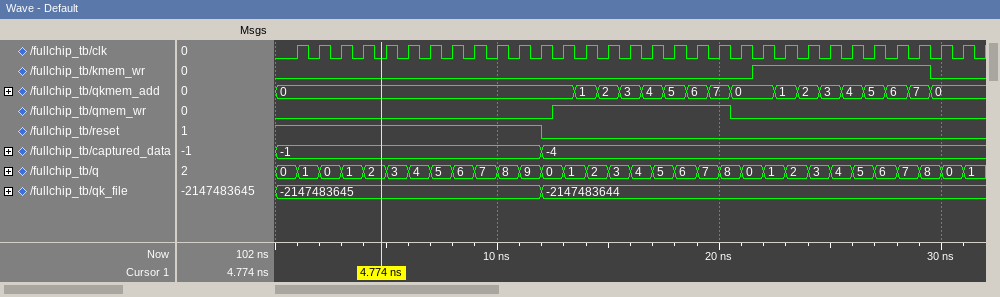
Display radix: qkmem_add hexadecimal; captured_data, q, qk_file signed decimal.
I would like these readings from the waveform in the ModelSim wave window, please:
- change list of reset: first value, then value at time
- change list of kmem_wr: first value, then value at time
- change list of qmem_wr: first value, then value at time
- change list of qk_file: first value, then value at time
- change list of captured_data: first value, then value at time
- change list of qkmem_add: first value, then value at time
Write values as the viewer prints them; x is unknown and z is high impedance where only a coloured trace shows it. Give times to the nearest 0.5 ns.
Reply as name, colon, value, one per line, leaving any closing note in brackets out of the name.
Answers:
change list of reset: first value, then value at time: 1, 0 at 12 ns
change list of kmem_wr: first value, then value at time: 0, 1 at 21.5 ns, 0 at 29.5 ns
change list of qmem_wr: first value, then value at time: 0, 1 at 12.5 ns, 0 at 20.5 ns
change list of qk_file: first value, then value at time: -2147483645, -2147483644 at 12 ns
change list of captured_data: first value, then value at time: -1, -4 at 12 ns
change list of qkmem_add: first value, then value at time: 0, 1 at 13.5 ns, 2 at 14.5 ns, 3 at 15.5 ns, 4 at 16.5 ns, 5 at 17.5 ns, 6 at 18.5 ns, 7 at 19.5 ns, 0 at 20.5 ns, 1 at 22.5 ns, 2 at 23.5 ns, 3 at 24.5 ns, 4 at 25.5 ns, 5 at 26.5 ns, 6 at 27.5 ns, 7 at 28.5 ns, 0 at 29.5 ns
